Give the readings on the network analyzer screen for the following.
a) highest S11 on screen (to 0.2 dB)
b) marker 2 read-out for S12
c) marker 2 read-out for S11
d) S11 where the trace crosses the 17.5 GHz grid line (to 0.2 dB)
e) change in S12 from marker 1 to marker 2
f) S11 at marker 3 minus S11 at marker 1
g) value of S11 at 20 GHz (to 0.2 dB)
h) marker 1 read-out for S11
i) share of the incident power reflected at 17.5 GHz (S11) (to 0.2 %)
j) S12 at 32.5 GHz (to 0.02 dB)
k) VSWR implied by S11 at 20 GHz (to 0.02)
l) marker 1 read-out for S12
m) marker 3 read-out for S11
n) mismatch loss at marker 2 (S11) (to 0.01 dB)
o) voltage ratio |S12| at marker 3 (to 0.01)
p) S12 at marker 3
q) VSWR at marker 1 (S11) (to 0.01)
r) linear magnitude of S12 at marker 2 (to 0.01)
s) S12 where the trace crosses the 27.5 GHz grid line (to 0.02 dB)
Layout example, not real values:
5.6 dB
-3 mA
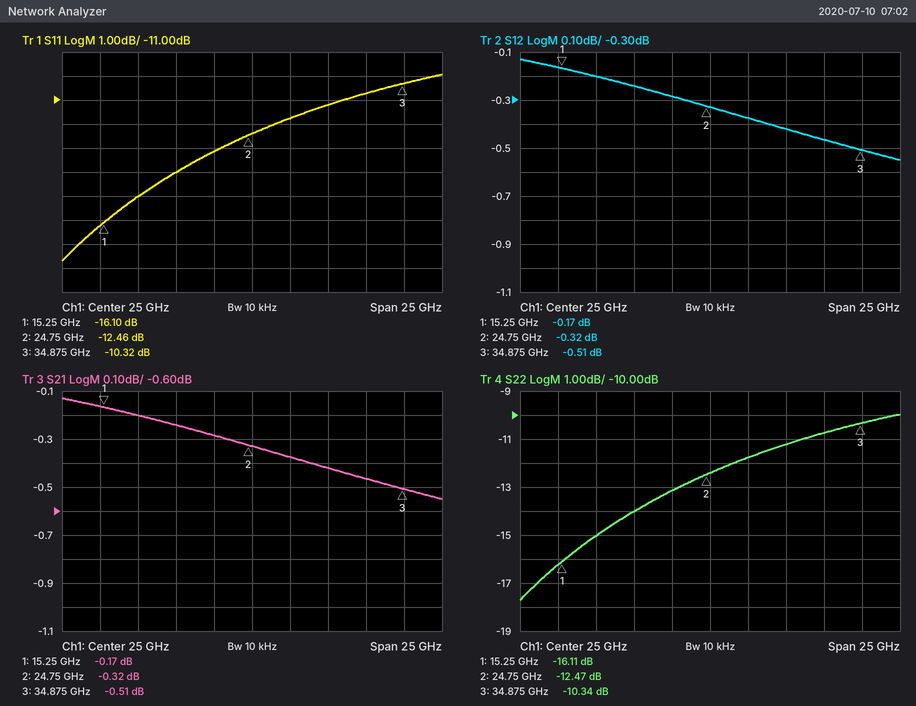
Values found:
-10.0 dB
-0.32 dB
-12.46 dB
-15.0 dB
-0.15 dB
5.78 dB
-14.0 dB
-16.10 dB
3.2 %
-0.46 dB
1.50
-0.17 dB
-10.32 dB
0.25 dB
0.94
-0.51 dB
1.37
0.96
-0.38 dB
